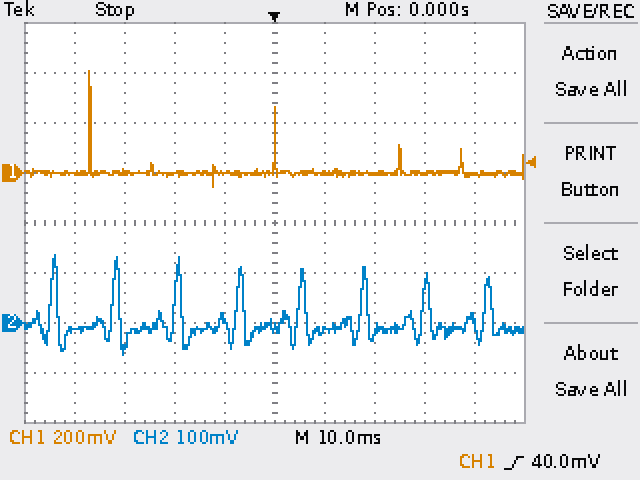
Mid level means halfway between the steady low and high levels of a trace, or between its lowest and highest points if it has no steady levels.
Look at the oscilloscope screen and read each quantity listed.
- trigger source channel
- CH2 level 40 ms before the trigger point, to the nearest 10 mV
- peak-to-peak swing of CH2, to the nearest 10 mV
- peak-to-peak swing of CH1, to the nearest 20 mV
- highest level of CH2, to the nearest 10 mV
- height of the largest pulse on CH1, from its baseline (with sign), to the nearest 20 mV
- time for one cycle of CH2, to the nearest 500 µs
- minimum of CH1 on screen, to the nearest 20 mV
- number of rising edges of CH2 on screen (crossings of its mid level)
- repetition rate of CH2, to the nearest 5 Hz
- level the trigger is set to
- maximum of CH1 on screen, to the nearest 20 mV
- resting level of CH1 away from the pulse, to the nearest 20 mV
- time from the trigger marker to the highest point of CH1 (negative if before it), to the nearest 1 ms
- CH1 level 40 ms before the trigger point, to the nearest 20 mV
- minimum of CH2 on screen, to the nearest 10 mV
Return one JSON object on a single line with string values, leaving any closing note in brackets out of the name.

{"trigger source channel": "CH1", "CH2 level 40 ms before the trigger point, to the nearest 10 mV": "-10 mV", "peak-to-peak swing of CH2, to the nearest 10 mV": "200 mV", "peak-to-peak swing of CH1, to the nearest 20 mV": "460 mV", "highest level of CH2, to the nearest 10 mV": "140 mV", "height of the largest pulse on CH1, from its baseline (with sign), to the nearest 20 mV": "+400 mV", "time for one cycle of CH2, to the nearest 500 µs": "12.5 ms", "minimum of CH1 on screen, to the nearest 20 mV": "-60 mV", "number of rising edges of CH2 on screen": "8", "repetition rate of CH2, to the nearest 5 Hz": "80 Hz", "level the trigger is set to": "40.0 mV", "maximum of CH1 on screen, to the nearest 20 mV": "400 mV", "resting level of CH1 away from the pulse, to the nearest 20 mV": "0 mV", "time from the trigger marker to the highest point of CH1 (negative if before it), to the nearest 1 ms": "-37 ms", "CH1 level 40 ms before the trigger point, to the nearest 20 mV": "0 mV", "minimum of CH2 on screen, to the nearest 10 mV": "-60 mV"}
